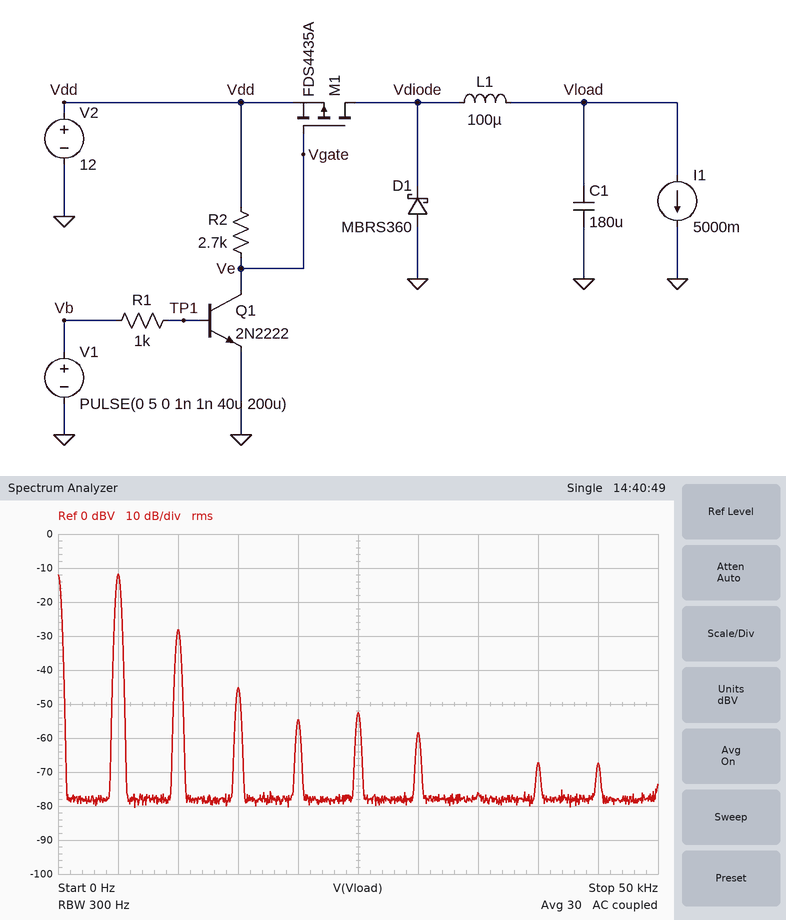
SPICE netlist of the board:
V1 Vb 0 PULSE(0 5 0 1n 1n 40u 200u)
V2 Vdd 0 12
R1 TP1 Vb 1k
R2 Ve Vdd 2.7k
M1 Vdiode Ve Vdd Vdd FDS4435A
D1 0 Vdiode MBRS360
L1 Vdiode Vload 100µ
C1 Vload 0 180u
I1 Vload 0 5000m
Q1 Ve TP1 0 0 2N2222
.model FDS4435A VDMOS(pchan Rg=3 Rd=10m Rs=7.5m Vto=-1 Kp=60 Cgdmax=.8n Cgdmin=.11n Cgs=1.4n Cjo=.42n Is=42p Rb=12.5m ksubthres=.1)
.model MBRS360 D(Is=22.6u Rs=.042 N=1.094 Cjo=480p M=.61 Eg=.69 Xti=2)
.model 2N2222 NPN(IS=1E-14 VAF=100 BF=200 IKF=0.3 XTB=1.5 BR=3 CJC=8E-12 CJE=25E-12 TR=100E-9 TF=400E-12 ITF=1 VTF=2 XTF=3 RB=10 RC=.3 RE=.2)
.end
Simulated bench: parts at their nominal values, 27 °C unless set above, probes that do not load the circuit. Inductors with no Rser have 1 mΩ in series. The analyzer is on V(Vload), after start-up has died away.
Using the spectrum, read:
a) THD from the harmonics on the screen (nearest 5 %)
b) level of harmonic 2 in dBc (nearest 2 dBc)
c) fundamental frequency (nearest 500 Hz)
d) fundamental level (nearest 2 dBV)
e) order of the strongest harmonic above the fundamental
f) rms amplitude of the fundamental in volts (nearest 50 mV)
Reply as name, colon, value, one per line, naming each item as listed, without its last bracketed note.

THD from the harmonics on the screen: 15 %
level of harmonic 2 in dBc: -16 dBc
fundamental frequency: 5.0 kHz
fundamental level: -12 dBV
order of the strongest harmonic above the fundamental: 2
rms amplitude of the fundamental in volts: 250 mV
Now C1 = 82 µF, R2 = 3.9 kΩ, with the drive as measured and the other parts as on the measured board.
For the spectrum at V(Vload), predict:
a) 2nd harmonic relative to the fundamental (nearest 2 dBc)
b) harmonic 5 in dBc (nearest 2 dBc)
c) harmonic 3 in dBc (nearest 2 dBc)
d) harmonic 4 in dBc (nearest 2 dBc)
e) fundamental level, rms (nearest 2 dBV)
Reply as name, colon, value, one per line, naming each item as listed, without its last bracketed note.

2nd harmonic relative to the fundamental: -18 dBc
harmonic 5 in dBc: -42 dBc
harmonic 3 in dBc: -44 dBc
harmonic 4 in dBc: -38 dBc
fundamental level, rms: -4 dBV
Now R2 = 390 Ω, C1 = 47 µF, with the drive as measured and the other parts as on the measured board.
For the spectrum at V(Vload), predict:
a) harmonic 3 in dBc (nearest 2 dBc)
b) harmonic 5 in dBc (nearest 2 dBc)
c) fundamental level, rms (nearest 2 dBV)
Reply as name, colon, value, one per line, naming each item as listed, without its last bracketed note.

harmonic 3 in dBc: -28 dBc
harmonic 5 in dBc: -54 dBc
fundamental level, rms: 0 dBV
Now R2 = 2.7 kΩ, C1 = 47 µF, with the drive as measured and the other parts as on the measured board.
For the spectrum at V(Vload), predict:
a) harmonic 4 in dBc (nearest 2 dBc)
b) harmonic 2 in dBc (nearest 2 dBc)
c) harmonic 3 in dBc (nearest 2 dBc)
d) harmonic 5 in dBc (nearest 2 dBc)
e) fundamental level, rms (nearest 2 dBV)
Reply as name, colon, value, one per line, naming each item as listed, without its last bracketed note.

harmonic 4 in dBc: -44 dBc
harmonic 2 in dBc: -18 dBc
harmonic 3 in dBc: -34 dBc
harmonic 5 in dBc: -42 dBc
fundamental level, rms: 2 dBV
